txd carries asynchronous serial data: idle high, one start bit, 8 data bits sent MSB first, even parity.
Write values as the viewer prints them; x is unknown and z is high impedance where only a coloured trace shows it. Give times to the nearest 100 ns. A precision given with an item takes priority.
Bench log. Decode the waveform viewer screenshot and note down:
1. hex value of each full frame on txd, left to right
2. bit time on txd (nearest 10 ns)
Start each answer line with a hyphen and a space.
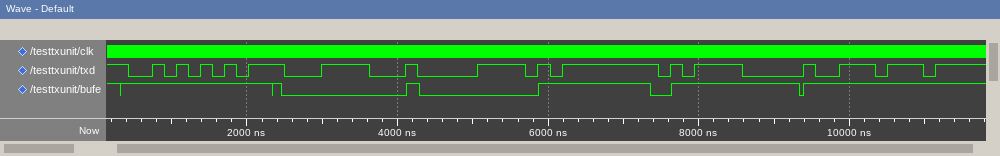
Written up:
- 55, 3C, 0F, FF, F0, 77
- 160 ns
